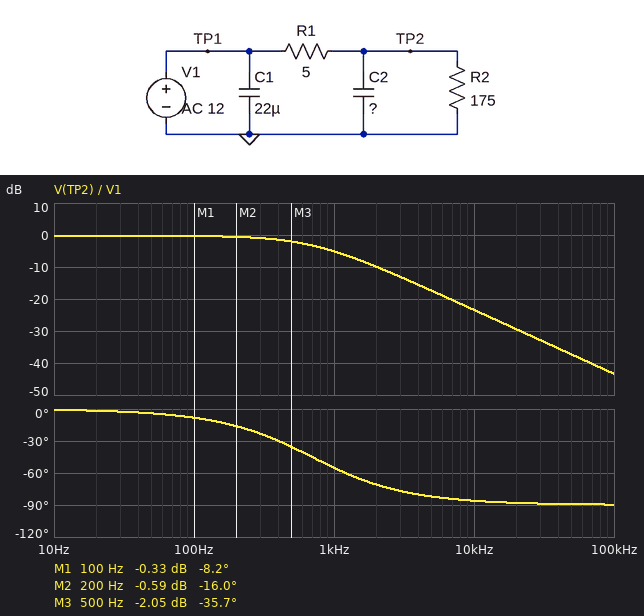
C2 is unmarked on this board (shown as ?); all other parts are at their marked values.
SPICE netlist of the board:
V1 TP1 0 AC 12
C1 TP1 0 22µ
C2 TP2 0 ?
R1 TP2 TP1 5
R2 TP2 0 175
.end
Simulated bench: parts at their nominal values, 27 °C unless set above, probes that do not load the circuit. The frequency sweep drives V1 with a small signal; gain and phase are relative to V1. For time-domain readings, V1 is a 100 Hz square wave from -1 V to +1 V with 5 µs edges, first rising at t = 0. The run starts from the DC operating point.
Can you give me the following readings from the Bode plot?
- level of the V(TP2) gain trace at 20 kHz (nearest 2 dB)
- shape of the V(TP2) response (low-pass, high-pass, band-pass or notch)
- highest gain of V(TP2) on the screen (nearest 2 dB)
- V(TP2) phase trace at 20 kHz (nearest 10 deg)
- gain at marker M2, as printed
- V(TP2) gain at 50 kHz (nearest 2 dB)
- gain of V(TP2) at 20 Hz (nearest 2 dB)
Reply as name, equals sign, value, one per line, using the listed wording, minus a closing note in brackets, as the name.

level of the V(TP2) gain trace at 20 kHz = -30 dB
shape of the V(TP2) response = low-pass
highest gain of V(TP2) on the screen = 0 dB
V(TP2) phase trace at 20 kHz = -90 deg
gain at marker M2, as printed = -0.59 dB
V(TP2) gain at 50 kHz = -38 dB
gain of V(TP2) at 20 Hz = 0 dB
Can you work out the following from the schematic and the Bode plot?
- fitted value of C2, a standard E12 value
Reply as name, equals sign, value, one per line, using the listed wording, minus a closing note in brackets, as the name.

fitted value of C2, a standard E12 value = 47 µF
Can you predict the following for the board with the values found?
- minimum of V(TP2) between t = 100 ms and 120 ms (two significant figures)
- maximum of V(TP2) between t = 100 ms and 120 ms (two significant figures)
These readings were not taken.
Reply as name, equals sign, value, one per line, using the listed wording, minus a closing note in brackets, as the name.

minimum of V(TP2) between t = 100 ms and 120 ms = -970 mV
maximum of V(TP2) between t = 100 ms and 120 ms = 970 mV
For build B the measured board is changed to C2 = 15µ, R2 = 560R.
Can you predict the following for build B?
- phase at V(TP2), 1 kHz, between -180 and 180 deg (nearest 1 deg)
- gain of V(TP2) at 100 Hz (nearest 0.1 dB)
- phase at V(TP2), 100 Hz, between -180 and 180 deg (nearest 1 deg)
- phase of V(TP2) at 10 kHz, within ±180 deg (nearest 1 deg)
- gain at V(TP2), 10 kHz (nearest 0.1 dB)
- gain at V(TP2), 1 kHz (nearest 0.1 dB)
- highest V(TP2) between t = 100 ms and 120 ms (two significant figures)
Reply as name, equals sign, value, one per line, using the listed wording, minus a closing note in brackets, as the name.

phase at V(TP2), 1 kHz, between -180 and 180 deg = -25 deg
gain of V(TP2) at 100 Hz = -0.1 dB
phase at V(TP2), 100 Hz, between -180 and 180 deg = -3 deg
phase of V(TP2) at 10 kHz, within ±180 deg = -78 deg
gain at V(TP2), 10 kHz = -13.7 dB
gain at V(TP2), 1 kHz = -0.9 dB
highest V(TP2) between t = 100 ms and 120 ms = 990 mV
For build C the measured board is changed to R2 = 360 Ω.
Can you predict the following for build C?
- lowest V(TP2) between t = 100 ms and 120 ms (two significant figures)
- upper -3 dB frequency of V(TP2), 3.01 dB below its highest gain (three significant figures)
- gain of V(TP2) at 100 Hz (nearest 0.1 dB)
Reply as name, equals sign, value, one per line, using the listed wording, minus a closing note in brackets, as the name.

lowest V(TP2) between t = 100 ms and 120 ms = -990 mV
upper -3 dB frequency of V(TP2), 3.01 dB below its highest gain = 687 Hz
gain of V(TP2) at 100 Hz = -0.2 dB
